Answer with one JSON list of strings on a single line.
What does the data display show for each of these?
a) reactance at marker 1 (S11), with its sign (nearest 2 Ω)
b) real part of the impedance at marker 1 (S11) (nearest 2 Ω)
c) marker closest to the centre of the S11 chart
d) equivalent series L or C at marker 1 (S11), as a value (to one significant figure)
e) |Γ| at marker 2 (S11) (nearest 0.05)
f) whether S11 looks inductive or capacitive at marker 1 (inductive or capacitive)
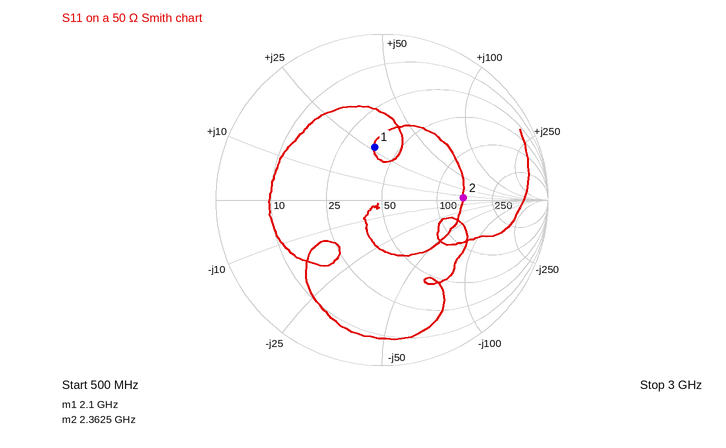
["+26 Ω", "38 Ω", "marker 1", "2 nH", "0.50", "inductive"]
